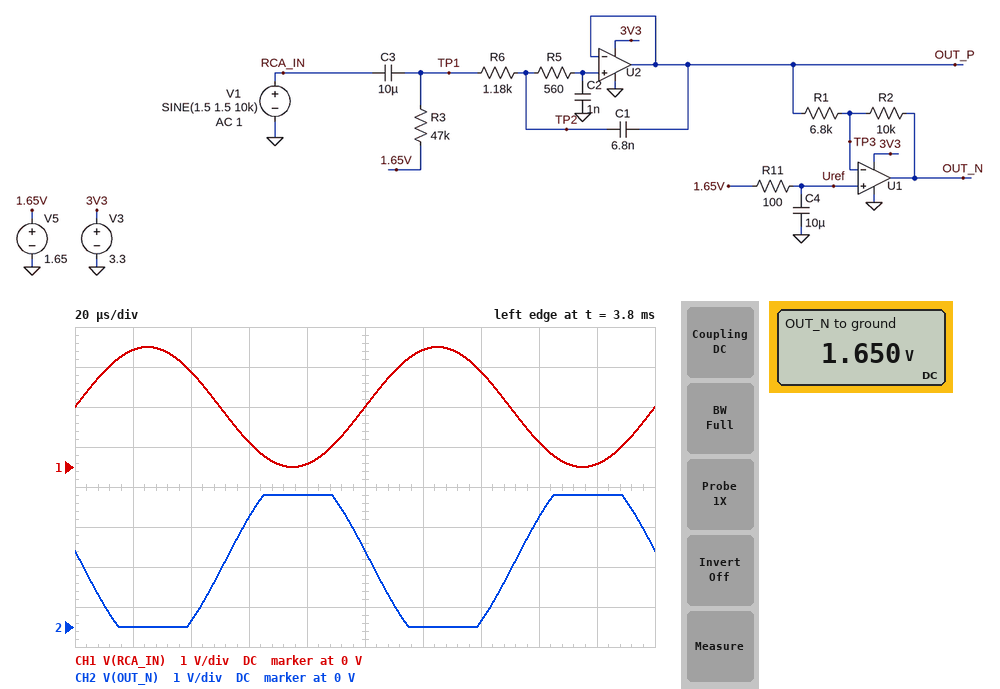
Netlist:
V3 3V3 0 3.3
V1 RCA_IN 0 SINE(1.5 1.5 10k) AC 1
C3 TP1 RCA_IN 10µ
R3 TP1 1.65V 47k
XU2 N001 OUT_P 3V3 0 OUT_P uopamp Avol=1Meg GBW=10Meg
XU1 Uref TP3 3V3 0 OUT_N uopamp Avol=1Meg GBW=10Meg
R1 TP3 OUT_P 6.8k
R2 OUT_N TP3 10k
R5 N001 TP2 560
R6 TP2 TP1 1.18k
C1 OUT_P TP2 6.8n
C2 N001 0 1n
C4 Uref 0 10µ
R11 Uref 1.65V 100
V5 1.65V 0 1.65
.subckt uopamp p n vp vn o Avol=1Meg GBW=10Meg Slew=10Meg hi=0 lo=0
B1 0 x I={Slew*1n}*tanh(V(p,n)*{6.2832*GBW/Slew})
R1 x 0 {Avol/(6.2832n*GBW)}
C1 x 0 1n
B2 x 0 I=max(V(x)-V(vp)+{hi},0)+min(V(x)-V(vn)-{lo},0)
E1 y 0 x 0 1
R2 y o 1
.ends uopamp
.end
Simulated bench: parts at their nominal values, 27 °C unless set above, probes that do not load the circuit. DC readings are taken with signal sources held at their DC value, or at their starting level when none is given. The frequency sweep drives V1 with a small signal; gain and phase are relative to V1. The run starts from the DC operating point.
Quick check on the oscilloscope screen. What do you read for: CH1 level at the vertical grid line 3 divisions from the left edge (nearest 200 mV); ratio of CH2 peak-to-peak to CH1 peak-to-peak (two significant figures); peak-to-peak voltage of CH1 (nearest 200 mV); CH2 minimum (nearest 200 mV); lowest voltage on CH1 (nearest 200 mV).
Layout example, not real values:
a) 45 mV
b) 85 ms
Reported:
a) 600 mV
b) 1.1
c) 3.0 V
d) 0 V
e) 0 V
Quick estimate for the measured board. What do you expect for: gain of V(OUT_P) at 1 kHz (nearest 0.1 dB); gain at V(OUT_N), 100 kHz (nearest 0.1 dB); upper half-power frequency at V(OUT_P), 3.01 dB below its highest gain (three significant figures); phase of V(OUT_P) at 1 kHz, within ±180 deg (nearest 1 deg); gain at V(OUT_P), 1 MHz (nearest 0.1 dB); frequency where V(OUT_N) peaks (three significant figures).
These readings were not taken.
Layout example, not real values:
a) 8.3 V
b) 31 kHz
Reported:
a) 0 dB
b) 0.6 dB
c) 88.0 kHz
d) -1 deg
e) -45.3 dB
f) 60.7 kHz
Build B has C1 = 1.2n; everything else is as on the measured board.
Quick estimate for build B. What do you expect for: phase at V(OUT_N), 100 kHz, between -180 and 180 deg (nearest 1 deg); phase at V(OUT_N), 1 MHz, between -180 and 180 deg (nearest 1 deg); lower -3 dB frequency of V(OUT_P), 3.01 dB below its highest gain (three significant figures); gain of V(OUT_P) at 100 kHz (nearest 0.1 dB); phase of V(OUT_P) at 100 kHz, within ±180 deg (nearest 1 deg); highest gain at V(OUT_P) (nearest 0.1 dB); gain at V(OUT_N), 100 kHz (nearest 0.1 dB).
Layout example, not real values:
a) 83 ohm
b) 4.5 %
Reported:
a) 120 deg
b) 0 deg
c) 339 mHz
d) -2.2 dB
e) -59 deg
f) 0 dB
g) 1.2 dB
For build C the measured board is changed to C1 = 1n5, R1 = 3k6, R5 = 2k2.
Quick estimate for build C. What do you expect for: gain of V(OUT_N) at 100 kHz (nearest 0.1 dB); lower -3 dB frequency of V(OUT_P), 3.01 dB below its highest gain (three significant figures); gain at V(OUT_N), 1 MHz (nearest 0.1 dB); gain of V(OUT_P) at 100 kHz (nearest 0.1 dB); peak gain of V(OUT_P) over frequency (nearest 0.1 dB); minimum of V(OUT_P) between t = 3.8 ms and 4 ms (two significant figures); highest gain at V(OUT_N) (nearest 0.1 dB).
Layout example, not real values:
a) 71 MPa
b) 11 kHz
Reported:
a) 2.0 dB
b) 339 mHz
c) -35.6 dB
d) -6.8 dB
e) 0 dB
f) 160 mV
g) 8.9 dB
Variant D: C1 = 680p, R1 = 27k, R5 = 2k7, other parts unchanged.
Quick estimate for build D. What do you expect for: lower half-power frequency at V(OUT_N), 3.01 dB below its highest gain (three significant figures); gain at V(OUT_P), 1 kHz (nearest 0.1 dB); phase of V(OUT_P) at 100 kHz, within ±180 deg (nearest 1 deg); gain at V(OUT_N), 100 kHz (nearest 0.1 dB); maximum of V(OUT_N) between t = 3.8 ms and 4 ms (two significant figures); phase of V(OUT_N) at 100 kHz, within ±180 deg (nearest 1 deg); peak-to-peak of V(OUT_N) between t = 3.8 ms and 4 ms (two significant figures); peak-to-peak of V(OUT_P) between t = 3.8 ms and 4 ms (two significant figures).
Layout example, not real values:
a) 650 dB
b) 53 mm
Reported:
a) 339 mHz
b) 0 dB
c) -87 deg
d) -16.4 dB
e) 2.2 V
f) 92 deg
g) 1.1 V
h) 2.9 V
